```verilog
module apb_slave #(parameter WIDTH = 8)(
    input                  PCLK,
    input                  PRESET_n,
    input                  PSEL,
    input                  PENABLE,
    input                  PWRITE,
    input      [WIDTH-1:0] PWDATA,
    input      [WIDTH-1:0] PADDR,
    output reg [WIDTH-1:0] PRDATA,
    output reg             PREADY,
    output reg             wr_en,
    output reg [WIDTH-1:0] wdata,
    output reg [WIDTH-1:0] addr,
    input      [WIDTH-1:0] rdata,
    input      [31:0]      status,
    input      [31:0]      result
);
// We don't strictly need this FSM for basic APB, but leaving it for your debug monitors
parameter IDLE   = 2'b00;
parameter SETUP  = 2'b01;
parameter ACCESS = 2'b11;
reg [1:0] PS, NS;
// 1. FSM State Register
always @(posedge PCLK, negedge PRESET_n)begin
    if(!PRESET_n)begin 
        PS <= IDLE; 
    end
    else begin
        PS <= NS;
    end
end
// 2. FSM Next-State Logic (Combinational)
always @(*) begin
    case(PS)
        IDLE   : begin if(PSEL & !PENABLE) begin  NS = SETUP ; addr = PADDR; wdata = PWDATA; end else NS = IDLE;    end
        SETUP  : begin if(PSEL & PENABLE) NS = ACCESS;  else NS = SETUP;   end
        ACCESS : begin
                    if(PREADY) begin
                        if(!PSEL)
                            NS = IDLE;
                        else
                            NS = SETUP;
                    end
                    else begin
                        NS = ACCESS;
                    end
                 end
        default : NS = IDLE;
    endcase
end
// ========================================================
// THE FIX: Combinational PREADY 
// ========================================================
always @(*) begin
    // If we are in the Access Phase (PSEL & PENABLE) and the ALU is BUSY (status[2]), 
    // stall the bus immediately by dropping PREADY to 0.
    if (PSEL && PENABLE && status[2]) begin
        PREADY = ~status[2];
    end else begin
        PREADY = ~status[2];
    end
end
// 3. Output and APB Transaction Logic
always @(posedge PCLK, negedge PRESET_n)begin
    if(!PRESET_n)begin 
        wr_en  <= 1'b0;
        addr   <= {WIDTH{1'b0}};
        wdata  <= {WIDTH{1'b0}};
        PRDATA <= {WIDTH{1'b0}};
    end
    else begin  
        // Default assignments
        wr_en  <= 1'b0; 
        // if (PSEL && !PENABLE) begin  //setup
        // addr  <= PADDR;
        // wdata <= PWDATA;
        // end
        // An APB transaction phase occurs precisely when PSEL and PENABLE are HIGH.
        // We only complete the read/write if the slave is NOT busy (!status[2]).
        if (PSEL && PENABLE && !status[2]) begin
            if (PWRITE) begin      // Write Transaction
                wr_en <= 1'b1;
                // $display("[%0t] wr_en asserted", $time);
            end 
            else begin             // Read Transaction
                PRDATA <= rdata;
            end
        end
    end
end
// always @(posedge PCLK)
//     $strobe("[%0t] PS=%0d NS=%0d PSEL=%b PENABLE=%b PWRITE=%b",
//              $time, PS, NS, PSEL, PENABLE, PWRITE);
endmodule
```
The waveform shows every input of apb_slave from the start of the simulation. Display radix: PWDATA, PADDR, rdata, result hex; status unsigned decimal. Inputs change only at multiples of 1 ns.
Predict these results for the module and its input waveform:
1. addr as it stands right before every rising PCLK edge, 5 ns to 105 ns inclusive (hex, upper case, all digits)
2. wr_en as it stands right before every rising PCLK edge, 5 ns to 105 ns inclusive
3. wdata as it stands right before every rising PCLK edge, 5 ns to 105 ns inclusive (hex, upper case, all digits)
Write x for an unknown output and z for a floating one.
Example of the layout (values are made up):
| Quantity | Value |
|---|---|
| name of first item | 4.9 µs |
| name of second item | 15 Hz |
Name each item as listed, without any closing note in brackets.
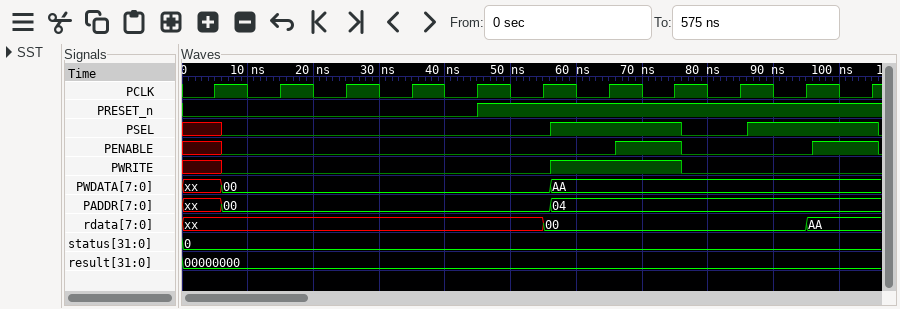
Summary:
| Quantity | Value |
|---|---|
| addr as it stands right before every rising PCLK edge, 5 ns to 105 ns inclusive | 00, 00, 00, 00, 00, 00, 04, 04, 04, 04, 04 |
| wr_en as it stands right before every rising PCLK edge, 5 ns to 105 ns inclusive | 0 0 0 0 0 0 0 0 1 0 0 |
| wdata as it stands right before every rising PCLK edge, 5 ns to 105 ns inclusive | 00, 00, 00, 00, 00, 00, AA, AA, AA, AA, AA |
